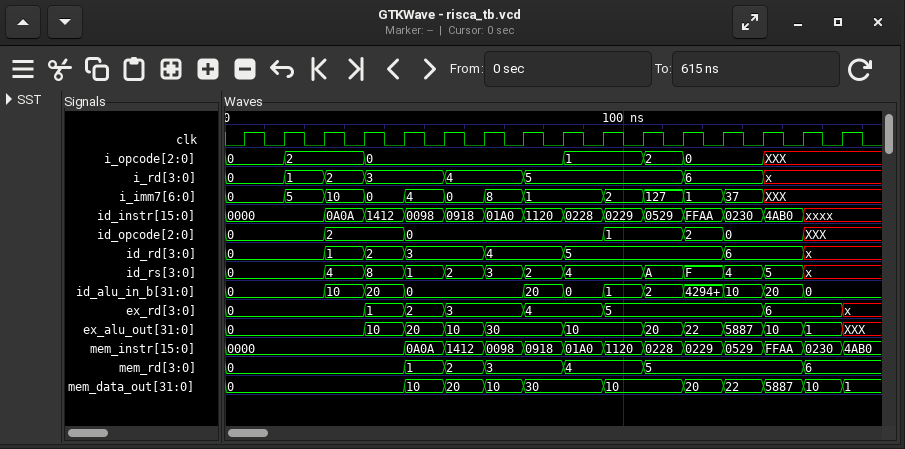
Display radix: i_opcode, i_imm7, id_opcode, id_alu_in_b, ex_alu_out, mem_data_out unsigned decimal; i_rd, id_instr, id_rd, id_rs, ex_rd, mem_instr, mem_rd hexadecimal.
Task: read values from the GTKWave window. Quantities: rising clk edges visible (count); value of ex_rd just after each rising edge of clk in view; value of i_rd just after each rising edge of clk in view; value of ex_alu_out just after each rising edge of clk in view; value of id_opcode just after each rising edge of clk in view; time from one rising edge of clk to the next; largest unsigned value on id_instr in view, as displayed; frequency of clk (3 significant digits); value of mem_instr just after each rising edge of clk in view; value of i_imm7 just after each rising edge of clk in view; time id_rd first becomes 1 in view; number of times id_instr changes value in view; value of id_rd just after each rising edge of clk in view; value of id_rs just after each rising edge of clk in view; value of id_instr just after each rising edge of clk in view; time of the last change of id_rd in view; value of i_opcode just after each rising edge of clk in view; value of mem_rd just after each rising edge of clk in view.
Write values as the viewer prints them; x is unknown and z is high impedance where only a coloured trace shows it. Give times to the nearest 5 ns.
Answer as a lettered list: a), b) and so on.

a) 16
b) 0, 0, 0, 1, 2, 3, 3, 4, 4, 5, 5, 5, 5, 6, 6, x
c) 0, 1, 2, 3, 3, 4, 4, 5, 5, 5, 5, 6, 6, x, x, x
d) 0, 0, 0, 10, 20, 10, 30, 30, 10, 10, 20, 22, 5887, 10, 1, XXX
e) 0, 0, 2, 2, 0, 0, 0, 0, 0, 1, 1, 2, 0, 0, XXX, XXX
f) 10 ns
g) FFAA
h) 100 MHz
i) 0000, 0000, 0000, 0000, 0A0A, 1412, 0098, 0918, 01A0, 1120, 0228, 0229, 0529, FFAA, 0230, 4AB0
j) 0, 5, 10, 0, 4, 0, 8, 1, 1, 2, 127, 1, 37, XXX, XXX, XXX
k) 25 ns
l) 13
m) 0, 0, 1, 2, 3, 3, 4, 4, 5, 5, 5, 5, 6, 6, x, x
n) 0, 0, 4, 8, 1, 2, 3, 2, 4, 4, A, F, 4, 5, x, x
o) 0000, 0000, 0A0A, 1412, 0098, 0918, 01A0, 1120, 0228, 0229, 0529, FFAA, 0230, 4AB0, xxxx, xxxx
p) 145 ns
q) 0, 2, 2, 0, 0, 0, 0, 0, 1, 1, 2, 0, 0, XXX, XXX, XXX
r) 0, 0, 0, 0, 1, 2, 3, 3, 4, 4, 5, 5, 5, 5, 6, 6
